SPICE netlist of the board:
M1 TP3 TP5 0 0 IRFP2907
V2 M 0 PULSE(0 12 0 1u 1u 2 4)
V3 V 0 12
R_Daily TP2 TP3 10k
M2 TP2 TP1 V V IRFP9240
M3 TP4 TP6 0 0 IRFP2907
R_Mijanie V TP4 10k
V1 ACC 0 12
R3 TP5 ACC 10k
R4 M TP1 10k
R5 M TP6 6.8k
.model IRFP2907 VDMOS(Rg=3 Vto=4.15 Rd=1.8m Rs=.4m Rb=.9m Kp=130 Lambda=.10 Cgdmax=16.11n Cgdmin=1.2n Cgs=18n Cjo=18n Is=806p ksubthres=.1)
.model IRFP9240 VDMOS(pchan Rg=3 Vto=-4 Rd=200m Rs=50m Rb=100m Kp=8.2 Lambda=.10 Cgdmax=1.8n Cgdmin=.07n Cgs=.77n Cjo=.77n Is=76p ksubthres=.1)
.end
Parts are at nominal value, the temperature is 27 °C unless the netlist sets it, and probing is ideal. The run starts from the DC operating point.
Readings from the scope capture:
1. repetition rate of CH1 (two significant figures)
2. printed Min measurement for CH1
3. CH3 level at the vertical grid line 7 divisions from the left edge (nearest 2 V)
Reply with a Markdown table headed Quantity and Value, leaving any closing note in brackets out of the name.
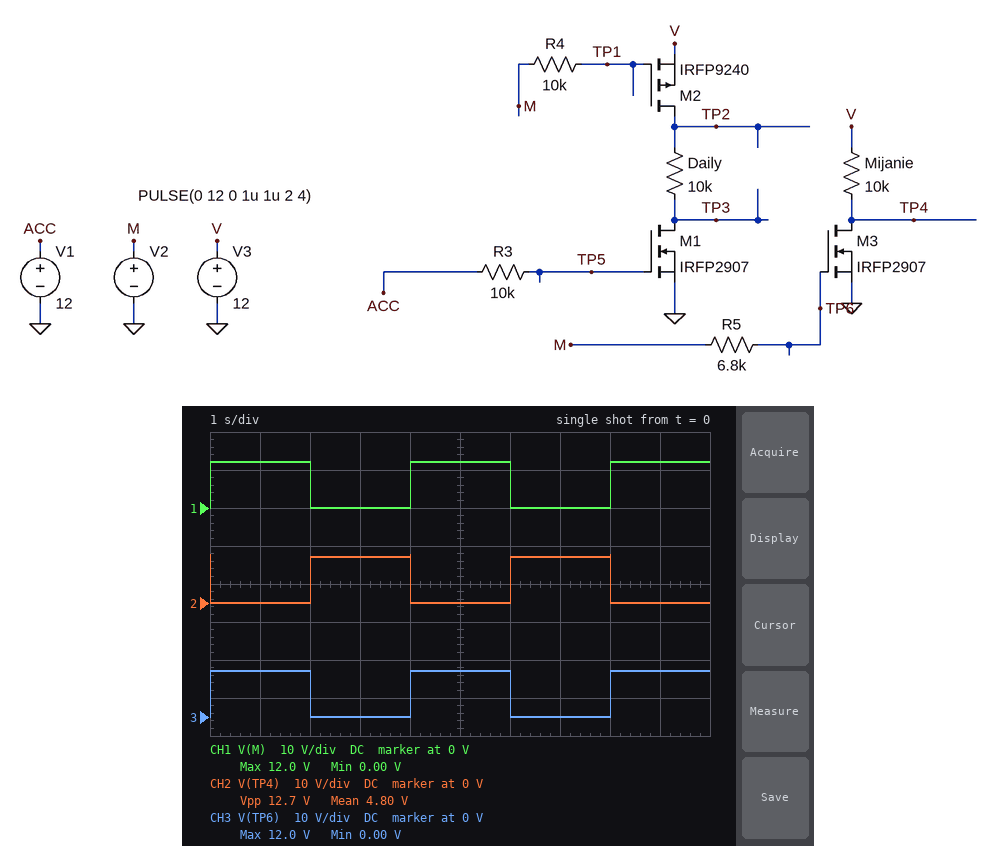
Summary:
| Quantity | Value |
|---|---|
| repetition rate of CH1 | 250 mHz |
| printed Min measurement for CH1 | 0.00 V |
| CH3 level at the vertical grid line 7 divisions from the left edge | 0 V |
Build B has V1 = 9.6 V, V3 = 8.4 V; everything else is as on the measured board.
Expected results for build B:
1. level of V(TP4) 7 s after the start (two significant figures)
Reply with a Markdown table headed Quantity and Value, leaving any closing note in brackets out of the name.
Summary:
| Quantity | Value |
|---|---|
| level of V(TP4) 7 s after the start | 8.4 V |
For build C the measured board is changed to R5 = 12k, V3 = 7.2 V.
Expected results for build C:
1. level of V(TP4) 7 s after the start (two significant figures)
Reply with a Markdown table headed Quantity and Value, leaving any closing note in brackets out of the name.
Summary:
| Quantity | Value |
|---|---|
| level of V(TP4) 7 s after the start | 7.2 V |
